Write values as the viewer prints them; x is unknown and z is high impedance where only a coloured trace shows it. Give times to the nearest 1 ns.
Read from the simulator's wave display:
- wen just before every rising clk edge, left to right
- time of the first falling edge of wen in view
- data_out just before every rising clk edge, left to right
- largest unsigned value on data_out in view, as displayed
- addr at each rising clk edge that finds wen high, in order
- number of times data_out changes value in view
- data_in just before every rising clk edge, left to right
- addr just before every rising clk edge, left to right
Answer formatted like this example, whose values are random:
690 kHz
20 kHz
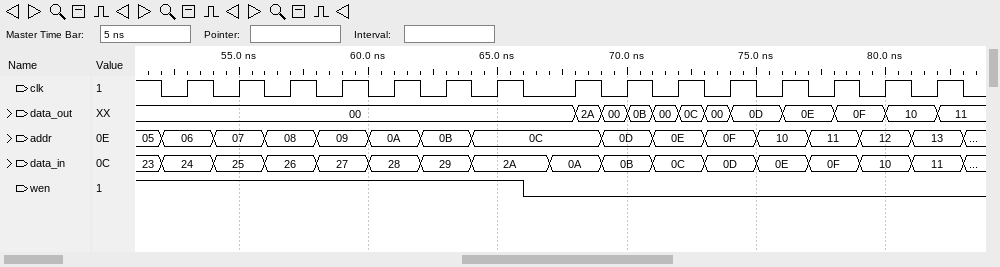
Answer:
1 1 1 1 1 1 1 0 0 0 0 0 0 0 0
66 ns
00, 00, 00, 00, 00, 00, 00, 00, 00, 00, 00, 0D, 0E, 0F, 10
2A
06, 07, 08, 09, 0A, 0B, 0C
11
24, 25, 26, 27, 28, 29, 2A, 0A, 0B, 0C, 0D, 0E, 0F, 10, 11
06, 07, 08, 09, 0A, 0B, 0C, 0C, 0D, 0E, 0F, 10, 11, 12, 13
